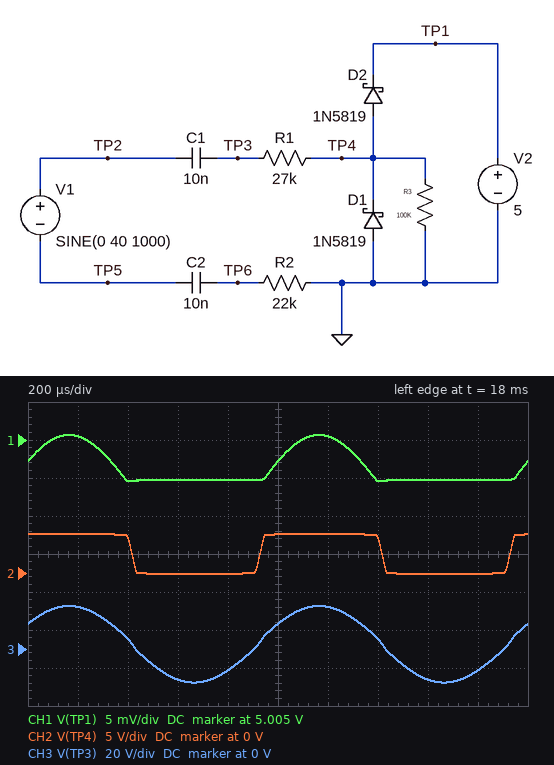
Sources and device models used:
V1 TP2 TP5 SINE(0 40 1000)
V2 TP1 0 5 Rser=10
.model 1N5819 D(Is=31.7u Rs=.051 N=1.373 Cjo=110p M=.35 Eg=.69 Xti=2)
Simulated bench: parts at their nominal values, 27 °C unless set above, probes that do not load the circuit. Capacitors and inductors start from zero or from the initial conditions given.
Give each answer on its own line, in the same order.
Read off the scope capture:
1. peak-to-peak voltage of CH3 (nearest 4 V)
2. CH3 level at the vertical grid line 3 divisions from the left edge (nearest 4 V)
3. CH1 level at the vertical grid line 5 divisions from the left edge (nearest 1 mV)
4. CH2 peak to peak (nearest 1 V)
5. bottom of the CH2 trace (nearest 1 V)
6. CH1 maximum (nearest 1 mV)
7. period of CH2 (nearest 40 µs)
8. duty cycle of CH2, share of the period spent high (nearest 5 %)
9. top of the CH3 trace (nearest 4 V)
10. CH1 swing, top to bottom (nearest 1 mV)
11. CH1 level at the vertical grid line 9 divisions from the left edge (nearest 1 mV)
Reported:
40 V
-16 V
5.002 V
5 V
0 V
5.006 V
1.00 ms
50 %
24 V
6 mV
5.000 V
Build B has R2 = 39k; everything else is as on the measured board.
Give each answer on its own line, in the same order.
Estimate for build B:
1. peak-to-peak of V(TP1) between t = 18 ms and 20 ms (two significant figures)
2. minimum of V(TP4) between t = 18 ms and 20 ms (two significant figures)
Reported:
4.7 mV
-99 mV
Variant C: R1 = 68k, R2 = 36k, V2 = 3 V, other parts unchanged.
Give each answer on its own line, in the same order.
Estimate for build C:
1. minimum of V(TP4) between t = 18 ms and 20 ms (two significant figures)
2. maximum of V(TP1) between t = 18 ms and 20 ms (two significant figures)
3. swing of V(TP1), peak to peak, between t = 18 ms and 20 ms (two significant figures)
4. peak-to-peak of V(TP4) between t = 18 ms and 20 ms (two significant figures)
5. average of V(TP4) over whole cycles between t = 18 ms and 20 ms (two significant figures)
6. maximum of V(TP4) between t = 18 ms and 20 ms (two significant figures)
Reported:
-86 mV
3.0 V
3.3 mV
3.2 V
1.5 V
3.1 V
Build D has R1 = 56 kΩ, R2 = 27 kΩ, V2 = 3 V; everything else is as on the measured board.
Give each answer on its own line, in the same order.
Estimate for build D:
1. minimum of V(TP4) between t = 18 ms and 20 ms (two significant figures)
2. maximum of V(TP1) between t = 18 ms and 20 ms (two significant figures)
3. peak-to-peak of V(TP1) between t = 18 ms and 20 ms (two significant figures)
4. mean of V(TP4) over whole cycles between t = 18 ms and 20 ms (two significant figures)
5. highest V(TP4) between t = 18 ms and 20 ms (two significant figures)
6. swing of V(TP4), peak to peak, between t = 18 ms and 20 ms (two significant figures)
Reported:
-93 mV
3.0 V
4.1 mV
1.5 V
3.1 V
3.2 V
